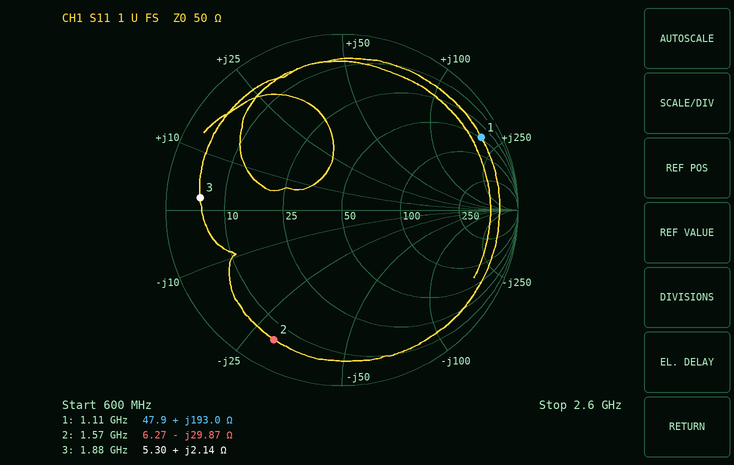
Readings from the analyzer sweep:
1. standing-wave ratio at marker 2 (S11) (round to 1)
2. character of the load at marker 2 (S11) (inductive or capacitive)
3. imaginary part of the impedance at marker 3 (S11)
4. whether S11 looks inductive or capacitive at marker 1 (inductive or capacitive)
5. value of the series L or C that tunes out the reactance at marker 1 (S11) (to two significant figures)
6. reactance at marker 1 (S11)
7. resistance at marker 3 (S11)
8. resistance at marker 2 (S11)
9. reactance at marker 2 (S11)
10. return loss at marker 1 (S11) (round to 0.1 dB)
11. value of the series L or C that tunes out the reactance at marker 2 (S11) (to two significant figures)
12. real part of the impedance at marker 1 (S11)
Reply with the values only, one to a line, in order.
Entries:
11
capacitive
+2.14 Ω
inductive
740 fF
+193.0 Ω
5.30 Ω
6.27 Ω
-29.87 Ω
1.0 dB
3.0 nH
47.9 Ω
